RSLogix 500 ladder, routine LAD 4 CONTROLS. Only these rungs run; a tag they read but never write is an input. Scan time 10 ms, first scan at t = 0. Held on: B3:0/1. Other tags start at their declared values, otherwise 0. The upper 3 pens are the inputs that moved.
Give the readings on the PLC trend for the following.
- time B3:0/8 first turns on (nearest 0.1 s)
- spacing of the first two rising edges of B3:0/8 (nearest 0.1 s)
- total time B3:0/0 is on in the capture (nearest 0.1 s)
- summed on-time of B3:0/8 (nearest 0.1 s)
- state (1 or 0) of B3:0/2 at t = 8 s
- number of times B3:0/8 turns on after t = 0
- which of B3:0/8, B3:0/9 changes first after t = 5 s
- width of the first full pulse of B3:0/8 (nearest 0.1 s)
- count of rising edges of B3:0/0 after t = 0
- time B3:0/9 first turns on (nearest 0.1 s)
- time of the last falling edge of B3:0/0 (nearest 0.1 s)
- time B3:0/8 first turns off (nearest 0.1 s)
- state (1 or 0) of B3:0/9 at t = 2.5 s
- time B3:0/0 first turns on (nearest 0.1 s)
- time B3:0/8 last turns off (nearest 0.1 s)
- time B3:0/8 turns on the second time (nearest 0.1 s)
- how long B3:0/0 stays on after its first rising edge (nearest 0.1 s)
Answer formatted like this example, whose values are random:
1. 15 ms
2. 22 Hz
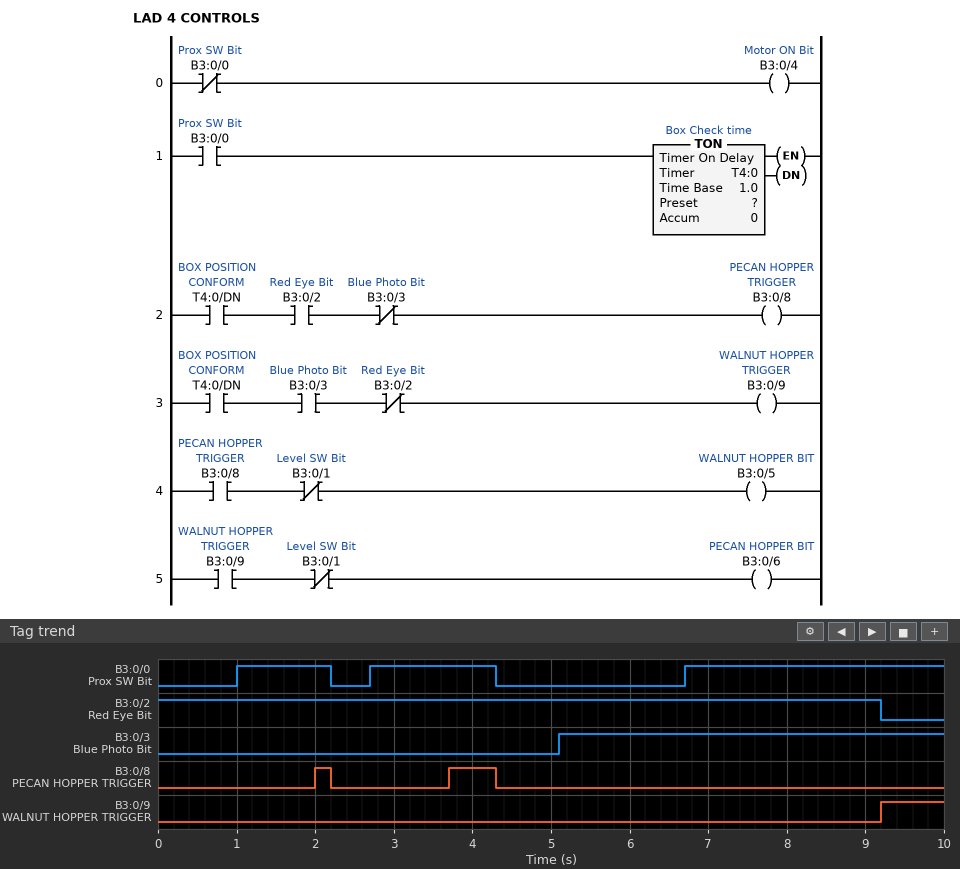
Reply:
1. 2.0 s
2. 1.7 s
3. 6.1 s
4. 0.8 s
5. 1
6. 2
7. B3:0/9
8. 0.2 s
9. 3
10. 9.2 s
11. 4.3 s
12. 2.2 s
13. 0
14. 1.0 s
15. 4.3 s
16. 3.7 s
17. 1.2 s
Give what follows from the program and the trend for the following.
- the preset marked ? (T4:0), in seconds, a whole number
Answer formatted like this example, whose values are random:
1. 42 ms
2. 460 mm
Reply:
1. 1 s
